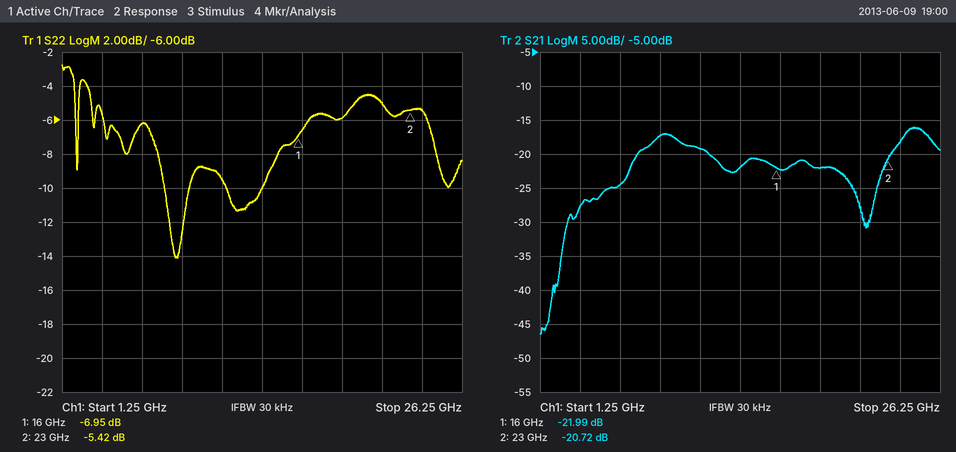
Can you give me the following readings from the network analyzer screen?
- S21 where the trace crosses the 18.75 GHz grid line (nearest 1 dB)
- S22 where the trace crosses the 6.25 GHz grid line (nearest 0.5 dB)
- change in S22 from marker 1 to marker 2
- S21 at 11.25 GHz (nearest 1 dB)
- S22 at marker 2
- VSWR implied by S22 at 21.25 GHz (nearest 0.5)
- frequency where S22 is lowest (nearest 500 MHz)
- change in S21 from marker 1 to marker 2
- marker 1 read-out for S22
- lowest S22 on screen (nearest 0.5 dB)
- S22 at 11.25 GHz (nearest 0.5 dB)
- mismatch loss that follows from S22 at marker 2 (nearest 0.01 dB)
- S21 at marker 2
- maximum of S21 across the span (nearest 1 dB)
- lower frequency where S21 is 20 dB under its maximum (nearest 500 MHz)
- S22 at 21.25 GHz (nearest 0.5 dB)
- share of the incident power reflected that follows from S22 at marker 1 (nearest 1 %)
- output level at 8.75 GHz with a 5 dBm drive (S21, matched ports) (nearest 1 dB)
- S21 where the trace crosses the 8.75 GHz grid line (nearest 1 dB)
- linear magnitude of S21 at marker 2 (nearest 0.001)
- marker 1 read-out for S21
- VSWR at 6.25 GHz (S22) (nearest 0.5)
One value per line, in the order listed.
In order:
-22 dB
-6.0 dB
1.53 dB
-19 dB
-5.42 dB
3.5
8.5 GHz
1.27 dB
-6.95 dB
-14.0 dB
-9.5 dB
1.47 dB
-20.72 dB
-16 dB
2.5 GHz
-5.0 dB
20 %
-12 dBm
-17 dB
0.092
-21.99 dB
3.0
